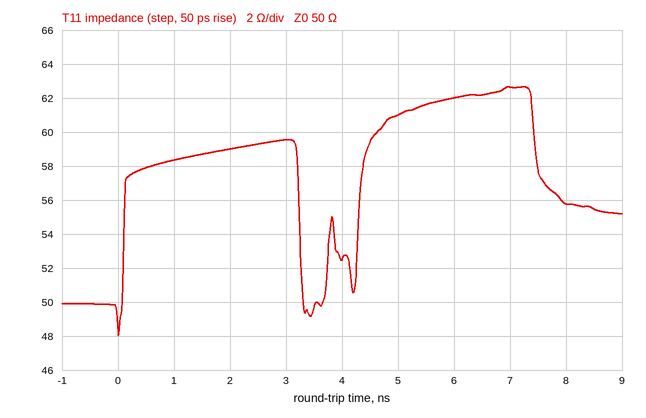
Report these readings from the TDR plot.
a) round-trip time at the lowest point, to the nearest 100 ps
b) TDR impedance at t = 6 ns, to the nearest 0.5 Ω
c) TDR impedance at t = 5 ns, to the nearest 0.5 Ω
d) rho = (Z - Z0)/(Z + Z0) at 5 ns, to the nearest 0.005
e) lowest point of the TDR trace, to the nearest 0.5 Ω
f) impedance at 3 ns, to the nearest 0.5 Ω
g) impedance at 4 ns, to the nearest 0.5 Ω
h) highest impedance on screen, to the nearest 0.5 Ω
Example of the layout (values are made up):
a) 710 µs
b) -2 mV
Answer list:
a) 0.0 ns
b) 62.0 Ω
c) 61.0 Ω
d) +0.100
e) 48.0 Ω
f) 59.5 Ω
g) 52.5 Ω
h) 62.5 Ω
